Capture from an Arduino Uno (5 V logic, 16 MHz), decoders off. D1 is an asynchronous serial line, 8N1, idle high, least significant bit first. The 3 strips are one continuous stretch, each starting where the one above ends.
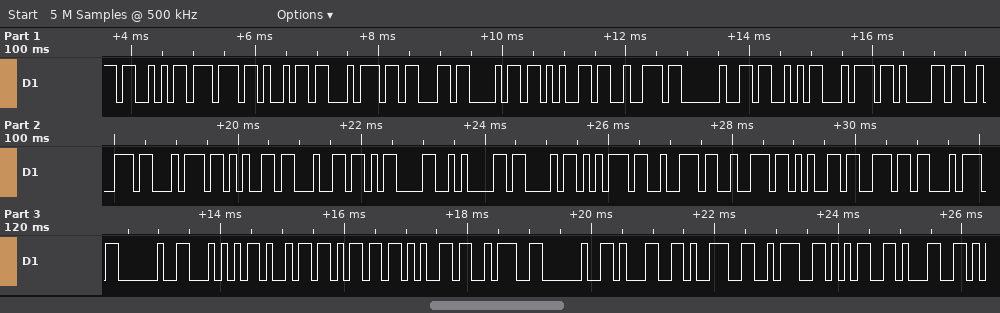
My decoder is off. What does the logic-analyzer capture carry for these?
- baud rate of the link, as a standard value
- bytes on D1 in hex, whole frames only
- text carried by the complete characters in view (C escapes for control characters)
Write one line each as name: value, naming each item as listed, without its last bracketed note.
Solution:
baud rate of the link, as a standard value: 9600 baud
bytes on D1 in hex, whole frames only: 53 77 69 74 63 68 65 72 20 53 74 61 72 74 65 64 0D 0A 43 75 72 72 65 6E 74 20 54 69 6D 65 3A 20 31 39 3A 35 31
text carried by the complete characters in view: "Switcher Started\r\nCurrent Time: 19:51"
